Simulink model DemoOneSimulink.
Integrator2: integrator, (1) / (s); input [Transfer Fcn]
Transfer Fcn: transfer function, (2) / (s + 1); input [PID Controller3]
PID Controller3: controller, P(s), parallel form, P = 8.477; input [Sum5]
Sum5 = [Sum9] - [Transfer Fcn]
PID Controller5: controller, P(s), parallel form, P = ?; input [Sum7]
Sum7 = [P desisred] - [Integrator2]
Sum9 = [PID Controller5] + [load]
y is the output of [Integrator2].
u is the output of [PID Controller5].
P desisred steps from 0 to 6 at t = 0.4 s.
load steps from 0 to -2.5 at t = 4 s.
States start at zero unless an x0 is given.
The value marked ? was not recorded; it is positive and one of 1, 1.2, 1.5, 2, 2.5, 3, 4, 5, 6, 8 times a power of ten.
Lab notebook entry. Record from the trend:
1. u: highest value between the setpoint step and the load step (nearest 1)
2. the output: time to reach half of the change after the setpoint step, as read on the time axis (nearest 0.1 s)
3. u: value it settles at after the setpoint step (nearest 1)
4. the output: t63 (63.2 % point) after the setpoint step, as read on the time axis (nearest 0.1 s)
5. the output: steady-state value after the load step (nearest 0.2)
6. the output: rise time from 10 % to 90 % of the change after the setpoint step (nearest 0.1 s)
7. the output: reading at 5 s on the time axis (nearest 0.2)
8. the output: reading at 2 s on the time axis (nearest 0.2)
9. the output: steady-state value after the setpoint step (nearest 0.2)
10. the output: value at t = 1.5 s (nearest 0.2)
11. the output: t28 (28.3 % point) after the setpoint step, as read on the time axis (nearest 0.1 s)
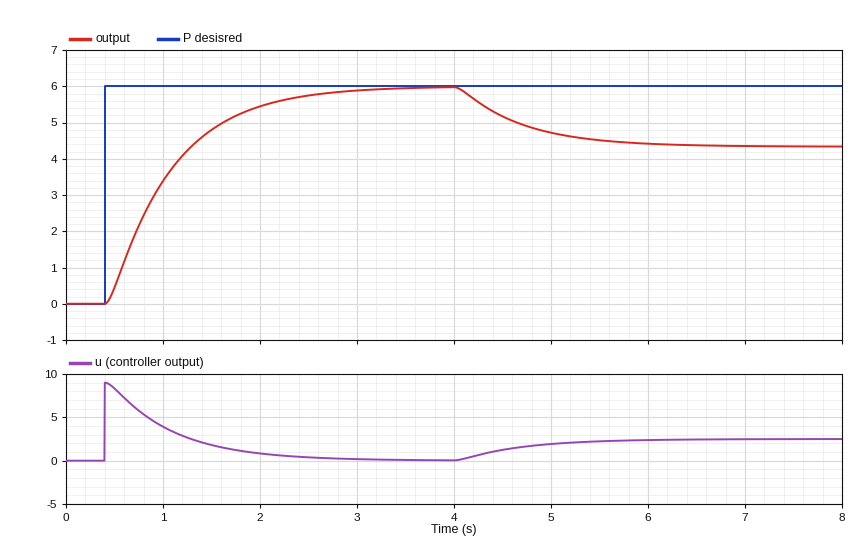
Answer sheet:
9
0.9 s
0
1.1 s
4.4
1.4 s
4.8
5.4
6.0
4.8
0.7 s
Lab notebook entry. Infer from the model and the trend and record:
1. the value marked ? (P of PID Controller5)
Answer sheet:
1.5
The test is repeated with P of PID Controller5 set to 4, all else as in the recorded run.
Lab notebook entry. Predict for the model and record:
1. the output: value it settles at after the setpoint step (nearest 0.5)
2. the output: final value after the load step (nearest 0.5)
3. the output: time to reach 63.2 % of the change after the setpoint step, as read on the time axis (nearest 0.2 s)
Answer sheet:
6.0
5.5
0.6 s
